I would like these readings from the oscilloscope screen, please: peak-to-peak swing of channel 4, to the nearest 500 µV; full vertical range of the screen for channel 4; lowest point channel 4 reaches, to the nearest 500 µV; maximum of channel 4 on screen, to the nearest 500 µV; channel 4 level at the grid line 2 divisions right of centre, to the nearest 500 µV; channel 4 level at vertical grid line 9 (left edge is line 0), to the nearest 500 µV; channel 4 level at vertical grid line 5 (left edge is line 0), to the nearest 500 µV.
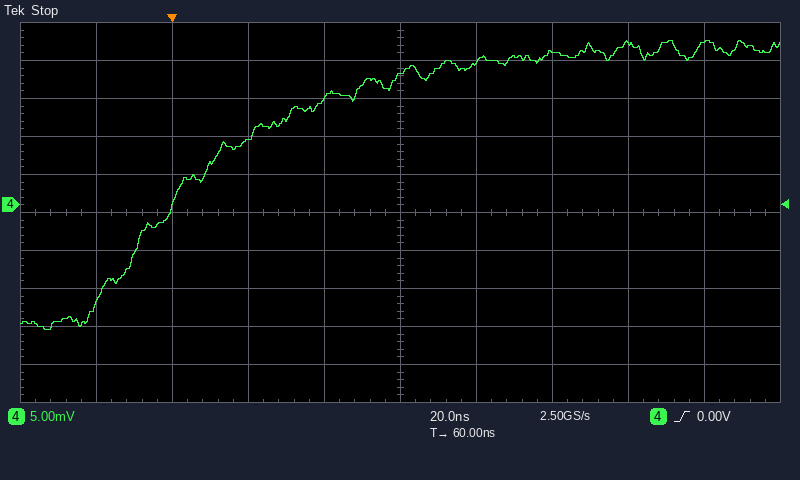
38.0 mV
50 mV
-16.5 mV
21.5 mV
20.0 mV
21.5 mV
17.0 mV
